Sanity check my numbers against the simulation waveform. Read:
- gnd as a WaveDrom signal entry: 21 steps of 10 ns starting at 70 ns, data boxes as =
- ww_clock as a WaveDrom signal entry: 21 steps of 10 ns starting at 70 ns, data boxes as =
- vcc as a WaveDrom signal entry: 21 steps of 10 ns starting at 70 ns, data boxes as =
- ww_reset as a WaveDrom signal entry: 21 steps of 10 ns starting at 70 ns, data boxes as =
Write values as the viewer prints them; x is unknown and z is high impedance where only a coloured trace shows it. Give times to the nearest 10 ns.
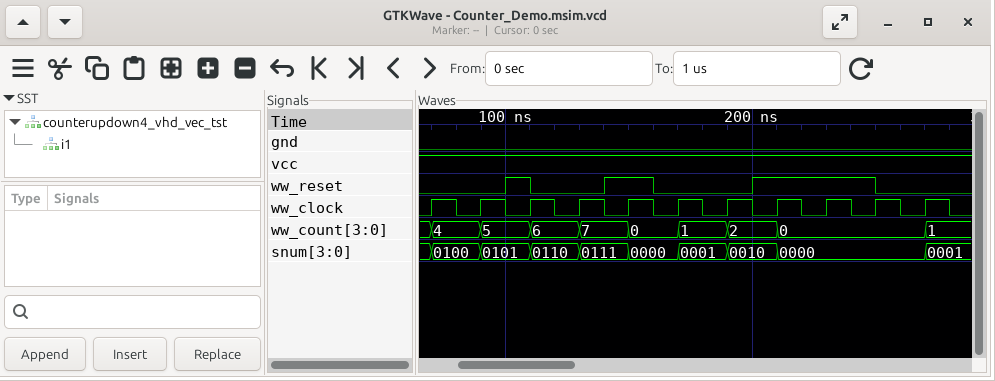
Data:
{name: 'gnd', wave: '0....................'}
{name: 'ww_clock', wave: '101010101010101010101'}
{name: 'vcc', wave: '1....................'}
{name: 'ww_reset', wave: '0..10..1.0...1....0..'}
